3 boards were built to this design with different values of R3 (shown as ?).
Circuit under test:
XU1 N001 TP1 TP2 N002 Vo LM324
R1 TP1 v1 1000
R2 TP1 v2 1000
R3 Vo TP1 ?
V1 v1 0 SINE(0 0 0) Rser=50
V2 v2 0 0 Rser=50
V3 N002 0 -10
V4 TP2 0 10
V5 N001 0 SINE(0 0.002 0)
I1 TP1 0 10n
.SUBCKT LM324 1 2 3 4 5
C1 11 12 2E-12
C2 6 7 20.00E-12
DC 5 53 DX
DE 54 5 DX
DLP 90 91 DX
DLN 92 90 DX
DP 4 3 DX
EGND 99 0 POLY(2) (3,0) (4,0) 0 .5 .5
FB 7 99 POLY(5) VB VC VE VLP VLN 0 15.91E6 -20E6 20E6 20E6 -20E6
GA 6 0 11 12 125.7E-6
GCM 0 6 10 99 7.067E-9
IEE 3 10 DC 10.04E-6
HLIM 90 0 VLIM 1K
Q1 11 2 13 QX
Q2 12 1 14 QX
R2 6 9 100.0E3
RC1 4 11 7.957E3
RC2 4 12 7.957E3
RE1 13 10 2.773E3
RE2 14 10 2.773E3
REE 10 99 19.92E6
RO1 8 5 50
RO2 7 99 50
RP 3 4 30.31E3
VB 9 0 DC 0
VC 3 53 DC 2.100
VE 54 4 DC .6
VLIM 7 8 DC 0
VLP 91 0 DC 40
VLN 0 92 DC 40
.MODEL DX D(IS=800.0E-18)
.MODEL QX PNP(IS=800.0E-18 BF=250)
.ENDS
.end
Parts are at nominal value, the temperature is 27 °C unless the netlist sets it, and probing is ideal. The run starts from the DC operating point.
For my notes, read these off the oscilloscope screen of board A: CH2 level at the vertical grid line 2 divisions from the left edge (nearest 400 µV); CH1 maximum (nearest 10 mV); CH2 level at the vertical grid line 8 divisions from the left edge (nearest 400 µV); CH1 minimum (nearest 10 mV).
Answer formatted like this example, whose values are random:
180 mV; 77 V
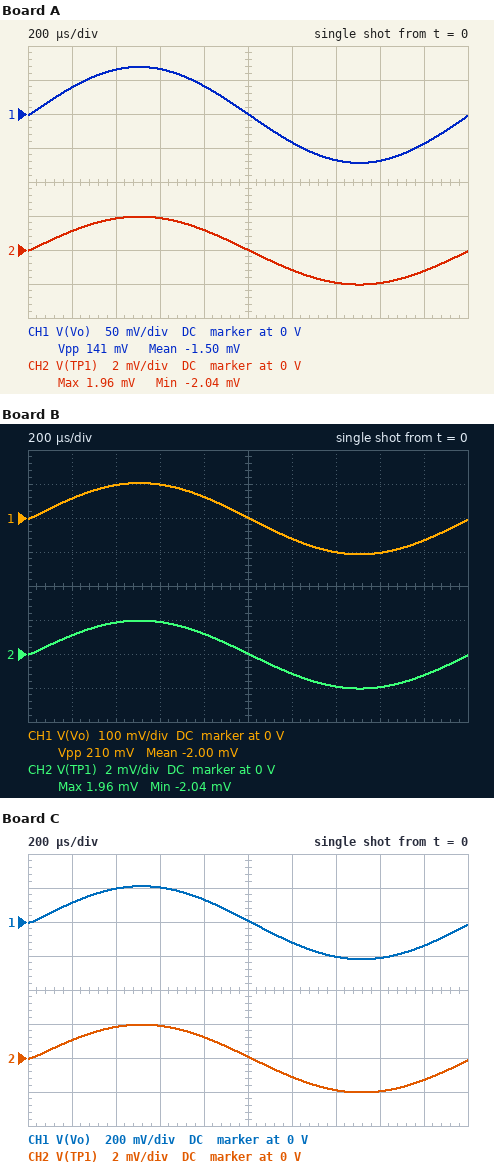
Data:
2.0 mV; 70 mV; -2.0 mV; -70 mV
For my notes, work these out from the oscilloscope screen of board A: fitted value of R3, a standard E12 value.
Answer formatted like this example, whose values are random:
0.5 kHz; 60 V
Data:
18 kΩ
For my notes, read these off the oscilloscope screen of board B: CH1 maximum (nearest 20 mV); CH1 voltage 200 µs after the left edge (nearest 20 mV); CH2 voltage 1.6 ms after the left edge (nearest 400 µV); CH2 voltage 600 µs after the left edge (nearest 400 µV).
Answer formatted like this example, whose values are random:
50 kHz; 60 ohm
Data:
100 mV; 60 mV; -2.0 mV; 2.0 mV
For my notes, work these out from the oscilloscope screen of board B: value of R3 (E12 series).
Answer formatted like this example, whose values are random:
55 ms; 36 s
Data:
27 kΩ
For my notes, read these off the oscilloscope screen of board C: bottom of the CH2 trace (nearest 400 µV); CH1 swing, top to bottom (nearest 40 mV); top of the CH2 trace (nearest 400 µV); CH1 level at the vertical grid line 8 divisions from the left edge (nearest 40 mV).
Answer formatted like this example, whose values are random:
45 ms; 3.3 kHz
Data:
-2.0 mV; 440 mV; 2.0 mV; -200 mV
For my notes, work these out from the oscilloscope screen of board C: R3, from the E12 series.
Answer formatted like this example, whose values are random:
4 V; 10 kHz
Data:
56 kΩ
